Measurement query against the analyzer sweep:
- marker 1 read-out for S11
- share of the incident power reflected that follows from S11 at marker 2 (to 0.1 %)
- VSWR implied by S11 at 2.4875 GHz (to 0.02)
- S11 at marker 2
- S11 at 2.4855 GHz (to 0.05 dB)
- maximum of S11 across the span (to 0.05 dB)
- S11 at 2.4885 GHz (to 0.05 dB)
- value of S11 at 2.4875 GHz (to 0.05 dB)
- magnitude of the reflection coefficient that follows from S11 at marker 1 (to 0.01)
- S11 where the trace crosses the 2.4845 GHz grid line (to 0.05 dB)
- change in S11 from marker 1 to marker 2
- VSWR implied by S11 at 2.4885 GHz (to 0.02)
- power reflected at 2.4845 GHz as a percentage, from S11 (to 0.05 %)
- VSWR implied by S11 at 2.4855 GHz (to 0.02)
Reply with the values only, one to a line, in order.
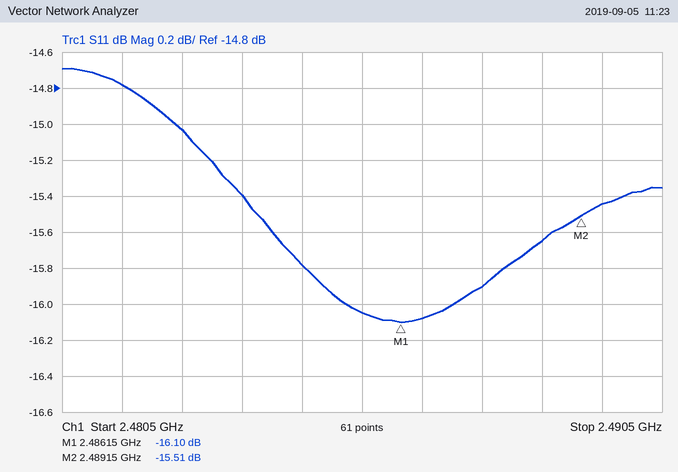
-16.10 dB
2.8 %
1.38
-15.51 dB
-16.05 dB
-14.70 dB
-15.65 dB
-15.90 dB
0.16
-15.80 dB
0.59 dB
1.40
2.65 %
1.38
